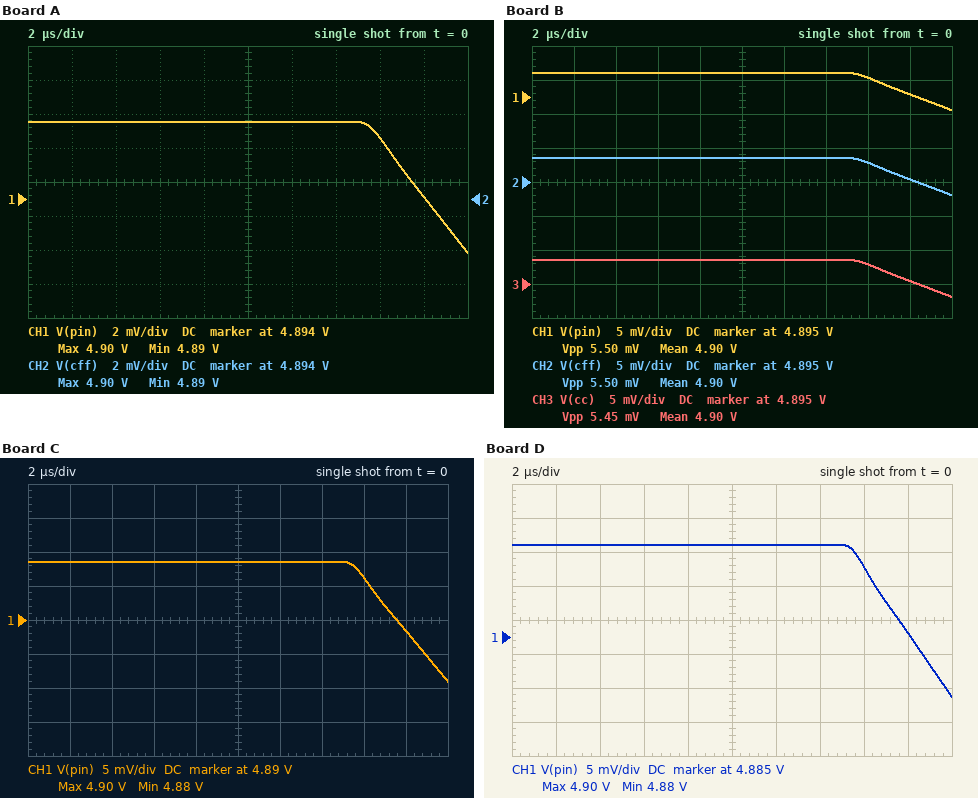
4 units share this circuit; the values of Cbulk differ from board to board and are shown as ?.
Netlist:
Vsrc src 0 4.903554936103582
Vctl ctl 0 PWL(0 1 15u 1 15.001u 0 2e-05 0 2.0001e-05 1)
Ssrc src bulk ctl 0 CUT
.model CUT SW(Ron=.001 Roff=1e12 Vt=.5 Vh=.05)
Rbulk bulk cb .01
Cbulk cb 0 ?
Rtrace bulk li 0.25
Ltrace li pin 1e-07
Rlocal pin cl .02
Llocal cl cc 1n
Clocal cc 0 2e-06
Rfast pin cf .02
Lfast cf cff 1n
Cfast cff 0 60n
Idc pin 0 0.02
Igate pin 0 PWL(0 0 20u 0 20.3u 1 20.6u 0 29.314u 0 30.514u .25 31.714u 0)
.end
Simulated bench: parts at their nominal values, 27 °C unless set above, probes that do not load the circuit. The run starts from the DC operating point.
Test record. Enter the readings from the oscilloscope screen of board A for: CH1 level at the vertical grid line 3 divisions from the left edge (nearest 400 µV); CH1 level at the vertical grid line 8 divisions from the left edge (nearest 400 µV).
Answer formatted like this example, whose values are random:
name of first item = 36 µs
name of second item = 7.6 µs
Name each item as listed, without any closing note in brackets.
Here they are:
CH1 level at the vertical grid line 3 divisions from the left edge = 4.8984 V
CH1 level at the vertical grid line 8 divisions from the left edge = 4.8976 V
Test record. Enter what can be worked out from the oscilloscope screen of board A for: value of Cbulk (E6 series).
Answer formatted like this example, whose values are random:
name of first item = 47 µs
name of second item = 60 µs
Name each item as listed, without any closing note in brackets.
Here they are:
value of Cbulk = 10 µF
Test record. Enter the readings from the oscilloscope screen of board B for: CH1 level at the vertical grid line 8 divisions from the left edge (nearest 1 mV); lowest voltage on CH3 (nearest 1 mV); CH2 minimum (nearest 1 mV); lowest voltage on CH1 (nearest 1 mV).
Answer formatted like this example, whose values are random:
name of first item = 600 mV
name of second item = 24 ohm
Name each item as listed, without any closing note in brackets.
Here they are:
CH1 level at the vertical grid line 8 divisions from the left edge = 4.898 V
lowest voltage on CH3 = 4.893 V
CH2 minimum = 4.893 V
lowest voltage on CH1 = 4.893 V
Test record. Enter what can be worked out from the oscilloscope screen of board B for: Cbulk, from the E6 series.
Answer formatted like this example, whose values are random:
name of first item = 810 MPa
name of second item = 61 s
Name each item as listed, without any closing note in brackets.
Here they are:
Cbulk, from the E6 series = 15 µF
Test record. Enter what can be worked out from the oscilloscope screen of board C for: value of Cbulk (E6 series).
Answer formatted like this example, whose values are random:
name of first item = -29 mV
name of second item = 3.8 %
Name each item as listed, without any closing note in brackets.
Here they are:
value of Cbulk = 3.3 µF
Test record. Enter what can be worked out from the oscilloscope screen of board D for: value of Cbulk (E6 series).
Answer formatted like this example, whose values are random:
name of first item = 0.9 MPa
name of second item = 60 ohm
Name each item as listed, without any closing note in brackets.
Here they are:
value of Cbulk = 2.2 µF
